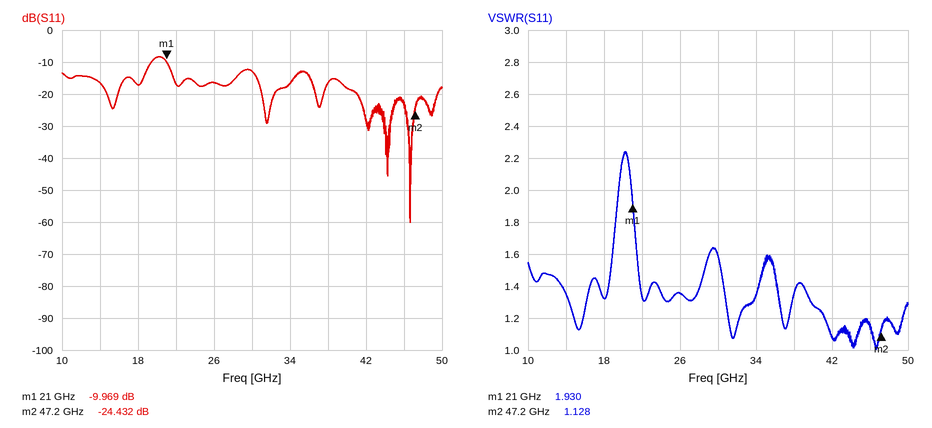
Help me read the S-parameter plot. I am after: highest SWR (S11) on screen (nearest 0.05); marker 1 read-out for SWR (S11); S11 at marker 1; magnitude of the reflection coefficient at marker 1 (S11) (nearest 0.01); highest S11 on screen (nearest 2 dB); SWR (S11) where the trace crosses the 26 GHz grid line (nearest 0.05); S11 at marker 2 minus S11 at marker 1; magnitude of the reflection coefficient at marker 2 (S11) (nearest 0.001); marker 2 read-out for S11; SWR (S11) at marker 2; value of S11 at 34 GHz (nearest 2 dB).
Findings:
2.25
1.930
-9.969 dB
0.32
-8 dB
1.35
-14.463 dB
0.060
-24.432 dB
1.128
-16 dB
